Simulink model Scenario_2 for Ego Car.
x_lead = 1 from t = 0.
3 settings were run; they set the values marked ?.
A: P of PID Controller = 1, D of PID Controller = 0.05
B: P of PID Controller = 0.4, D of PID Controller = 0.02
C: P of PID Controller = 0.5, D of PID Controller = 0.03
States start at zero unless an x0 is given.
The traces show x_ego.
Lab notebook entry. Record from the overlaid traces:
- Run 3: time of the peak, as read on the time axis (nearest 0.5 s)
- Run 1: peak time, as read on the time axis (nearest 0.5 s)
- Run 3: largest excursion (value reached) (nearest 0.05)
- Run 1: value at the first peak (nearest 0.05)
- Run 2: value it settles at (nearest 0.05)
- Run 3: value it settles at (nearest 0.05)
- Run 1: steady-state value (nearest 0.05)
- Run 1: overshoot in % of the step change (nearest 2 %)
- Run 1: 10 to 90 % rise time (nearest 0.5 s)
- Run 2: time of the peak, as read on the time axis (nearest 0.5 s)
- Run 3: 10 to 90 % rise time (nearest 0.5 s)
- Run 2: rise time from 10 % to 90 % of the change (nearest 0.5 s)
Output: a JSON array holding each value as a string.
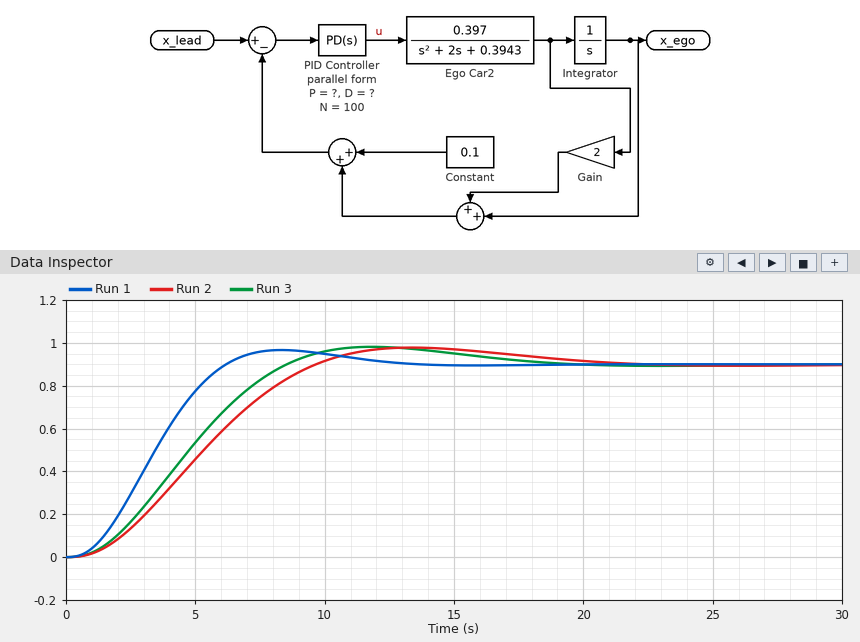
["12.0 s", "8.5 s", "1.00", "0.95", "0.90", "0.90", "0.90", "8 %", "4.0 s", "13.5 s", "5.5 s", "6.0 s"]
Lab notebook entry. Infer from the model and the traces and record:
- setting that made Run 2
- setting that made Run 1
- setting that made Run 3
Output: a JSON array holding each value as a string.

["B", "A", "C"]
